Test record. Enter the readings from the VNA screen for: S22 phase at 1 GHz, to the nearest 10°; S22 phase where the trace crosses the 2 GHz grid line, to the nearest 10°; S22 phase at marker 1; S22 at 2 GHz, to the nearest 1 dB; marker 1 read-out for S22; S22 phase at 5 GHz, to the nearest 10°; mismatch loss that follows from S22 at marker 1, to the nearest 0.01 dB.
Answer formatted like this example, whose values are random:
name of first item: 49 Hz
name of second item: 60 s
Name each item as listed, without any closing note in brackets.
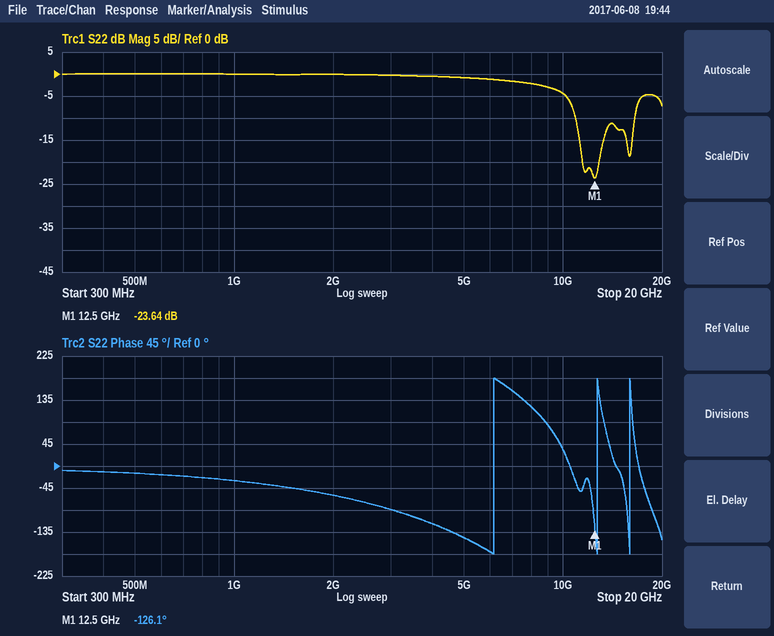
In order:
S22 phase at 1 GHz, to the nearest 10°: -30°
S22 phase where the trace crosses the 2 GHz grid line, to the nearest 10°: -60°
S22 phase at marker 1: -126.1°
S22 at 2 GHz, to the nearest 1 dB: 0 dB
marker 1 read-out for S22: -23.64 dB
S22 phase at 5 GHz, to the nearest 10°: -150°
mismatch loss that follows from S22 at marker 1, to the nearest 0.01 dB: 0.02 dB
